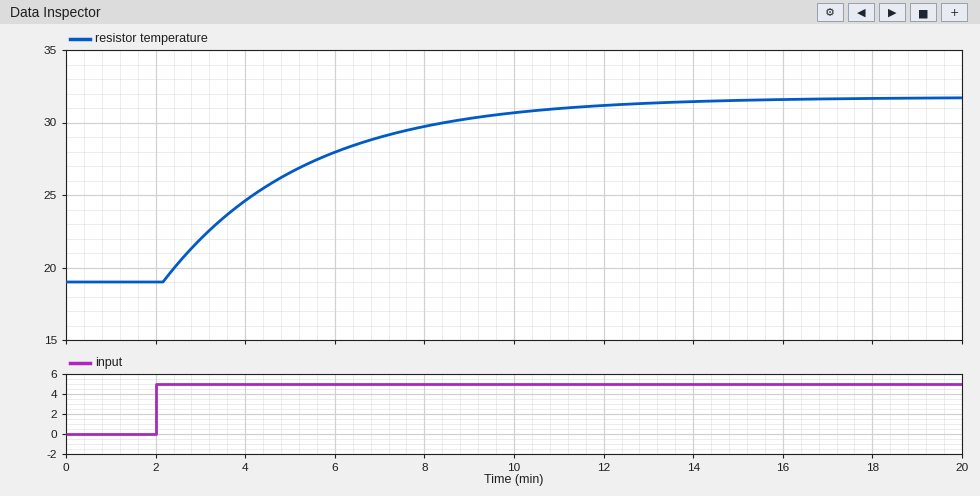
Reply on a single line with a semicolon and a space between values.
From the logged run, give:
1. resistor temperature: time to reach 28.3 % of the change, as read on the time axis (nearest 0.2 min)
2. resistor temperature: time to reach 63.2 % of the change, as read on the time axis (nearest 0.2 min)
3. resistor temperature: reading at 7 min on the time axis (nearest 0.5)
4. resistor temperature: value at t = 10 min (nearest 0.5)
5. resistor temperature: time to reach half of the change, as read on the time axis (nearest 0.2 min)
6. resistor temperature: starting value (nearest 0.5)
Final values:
3.2 min; 5.4 min; 29.0; 30.5; 4.4 min; 19.0
